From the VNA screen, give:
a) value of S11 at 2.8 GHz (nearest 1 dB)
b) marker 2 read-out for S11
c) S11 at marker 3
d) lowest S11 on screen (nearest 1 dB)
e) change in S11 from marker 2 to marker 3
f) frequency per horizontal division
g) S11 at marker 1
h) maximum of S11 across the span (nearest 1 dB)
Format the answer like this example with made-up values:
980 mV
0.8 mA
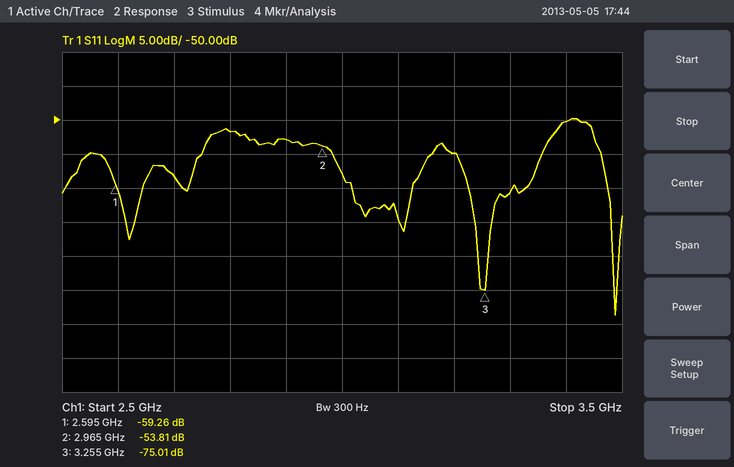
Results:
-52 dB
-53.81 dB
-75.01 dB
-79 dB
-21.20 dB
100 MHz
-59.26 dB
-50 dB
